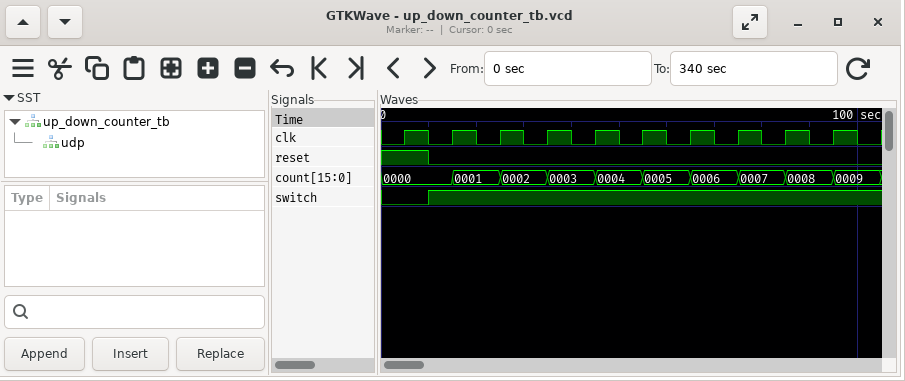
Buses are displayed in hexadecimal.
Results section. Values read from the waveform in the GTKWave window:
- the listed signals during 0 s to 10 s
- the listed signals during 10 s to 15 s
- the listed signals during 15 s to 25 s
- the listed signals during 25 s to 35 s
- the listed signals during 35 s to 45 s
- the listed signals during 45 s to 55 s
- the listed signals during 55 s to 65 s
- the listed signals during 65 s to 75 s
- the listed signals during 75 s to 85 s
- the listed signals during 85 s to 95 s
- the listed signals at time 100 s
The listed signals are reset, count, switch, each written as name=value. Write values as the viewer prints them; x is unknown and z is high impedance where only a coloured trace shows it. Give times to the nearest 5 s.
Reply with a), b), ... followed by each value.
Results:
a) reset=1, count=0000, switch=0
b) reset=0, count=0000, switch=1
c) reset=0, count=0001, switch=1
d) reset=0, count=0002, switch=1
e) reset=0, count=0003, switch=1
f) reset=0, count=0004, switch=1
g) reset=0, count=0005, switch=1
h) reset=0, count=0006, switch=1
i) reset=0, count=0007, switch=1
j) reset=0, count=0008, switch=1
k) reset=0, count=0009, switch=1
